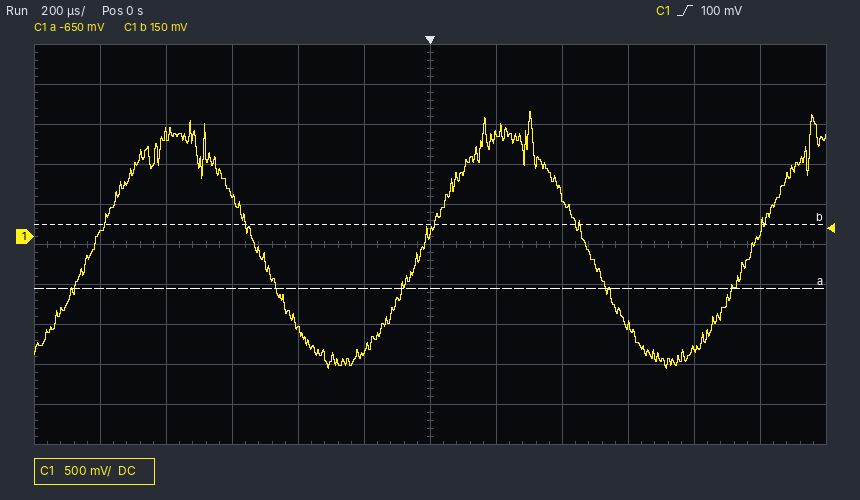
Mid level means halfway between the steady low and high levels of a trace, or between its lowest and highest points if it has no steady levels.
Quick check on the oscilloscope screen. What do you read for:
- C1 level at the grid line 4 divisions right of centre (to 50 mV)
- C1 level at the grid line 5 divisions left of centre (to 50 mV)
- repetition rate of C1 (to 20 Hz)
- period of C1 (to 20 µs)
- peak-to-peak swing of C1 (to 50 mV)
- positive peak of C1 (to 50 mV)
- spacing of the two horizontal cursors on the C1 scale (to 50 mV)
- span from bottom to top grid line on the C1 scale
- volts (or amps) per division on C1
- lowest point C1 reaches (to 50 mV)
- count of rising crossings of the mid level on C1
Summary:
-1.40 V
50 mV
1.00 kHz
1.00 ms
3.20 V
1.55 V
800 mV
5 V
500 mV
-1.65 V
3
